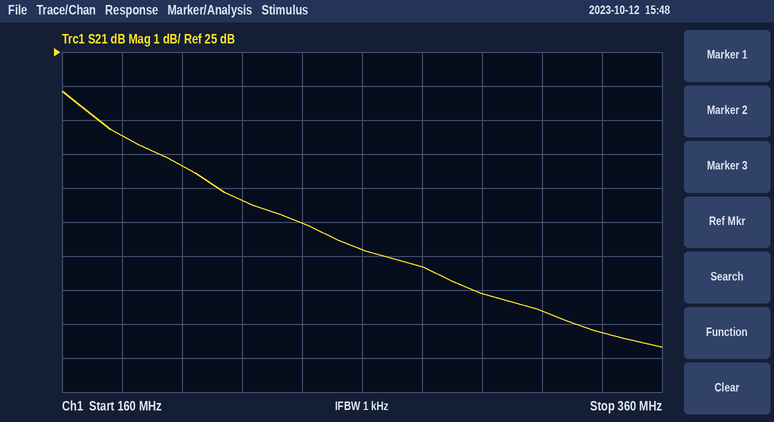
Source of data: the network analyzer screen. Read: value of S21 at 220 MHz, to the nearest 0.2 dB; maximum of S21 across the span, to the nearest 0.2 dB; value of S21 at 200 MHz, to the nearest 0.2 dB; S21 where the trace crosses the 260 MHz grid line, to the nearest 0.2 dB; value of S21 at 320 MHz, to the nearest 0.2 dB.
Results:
20.6 dB
23.8 dB
21.6 dB
19.2 dB
17.4 dB
